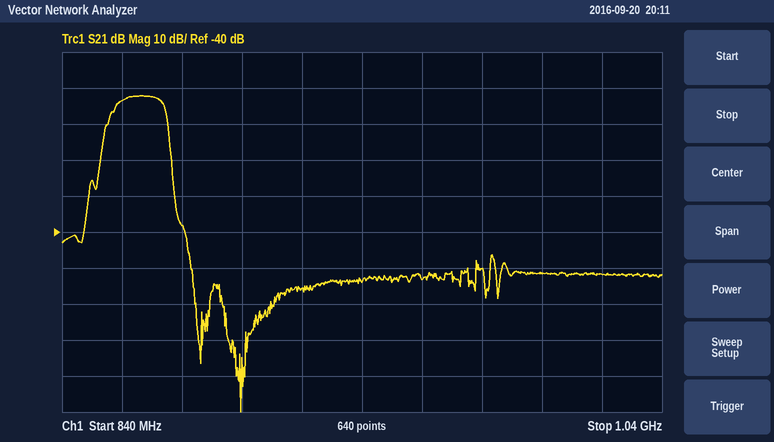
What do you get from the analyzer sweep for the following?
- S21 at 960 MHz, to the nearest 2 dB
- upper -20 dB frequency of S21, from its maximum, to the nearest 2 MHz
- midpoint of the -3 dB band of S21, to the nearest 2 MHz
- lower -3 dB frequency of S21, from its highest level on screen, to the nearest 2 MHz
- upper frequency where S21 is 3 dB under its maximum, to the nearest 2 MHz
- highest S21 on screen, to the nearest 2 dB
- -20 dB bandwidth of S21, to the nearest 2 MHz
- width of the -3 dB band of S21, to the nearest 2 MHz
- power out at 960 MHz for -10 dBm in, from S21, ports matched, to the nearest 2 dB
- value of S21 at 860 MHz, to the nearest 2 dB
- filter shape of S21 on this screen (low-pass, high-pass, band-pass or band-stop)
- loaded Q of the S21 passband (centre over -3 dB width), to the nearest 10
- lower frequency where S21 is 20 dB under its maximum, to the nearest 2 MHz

-54 dB
876 MHz
866 MHz
858 MHz
874 MHz
-2 dB
24 MHz
16 MHz
-64 dBm
-4 dB
band-pass
50
852 MHz
